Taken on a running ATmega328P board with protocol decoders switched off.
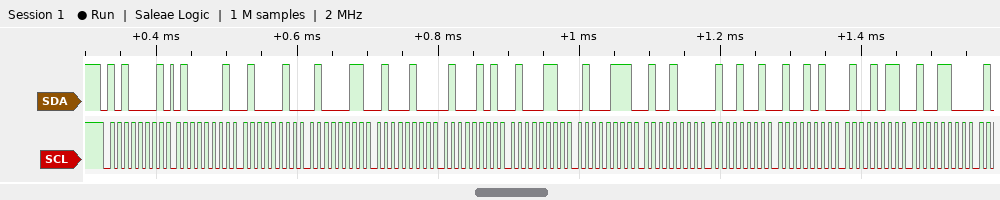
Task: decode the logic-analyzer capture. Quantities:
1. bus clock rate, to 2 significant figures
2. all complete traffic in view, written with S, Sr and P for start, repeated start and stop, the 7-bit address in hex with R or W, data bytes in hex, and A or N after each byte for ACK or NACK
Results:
100 kHz
S 50R A 41 A 42 A 43 A 44 A 45 A 46 A 47 A 48 A 49 A 4A A 4B A 4C A
